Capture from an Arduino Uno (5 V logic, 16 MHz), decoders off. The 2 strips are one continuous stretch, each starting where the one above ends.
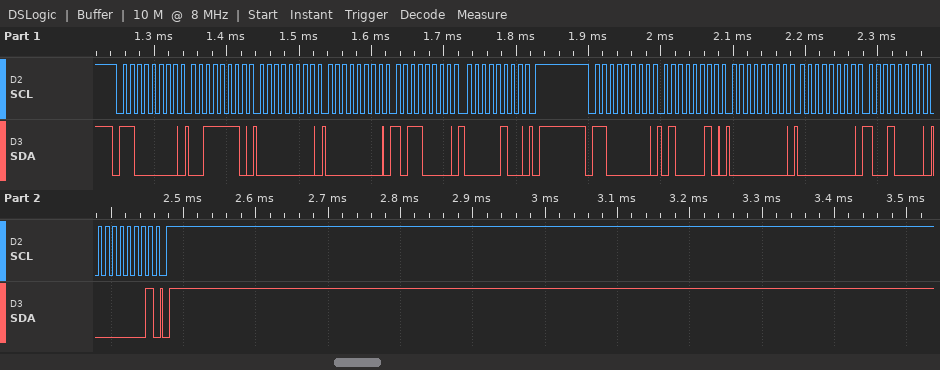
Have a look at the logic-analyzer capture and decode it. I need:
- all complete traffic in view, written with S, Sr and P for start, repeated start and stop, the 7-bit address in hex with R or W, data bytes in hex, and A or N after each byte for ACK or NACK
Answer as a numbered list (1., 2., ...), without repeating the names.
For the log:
1. S 60W A 3E A 00 A 00 A B0 A 04 A P S 60W A 42 A 00 A 00 A 90 A 01 A P
